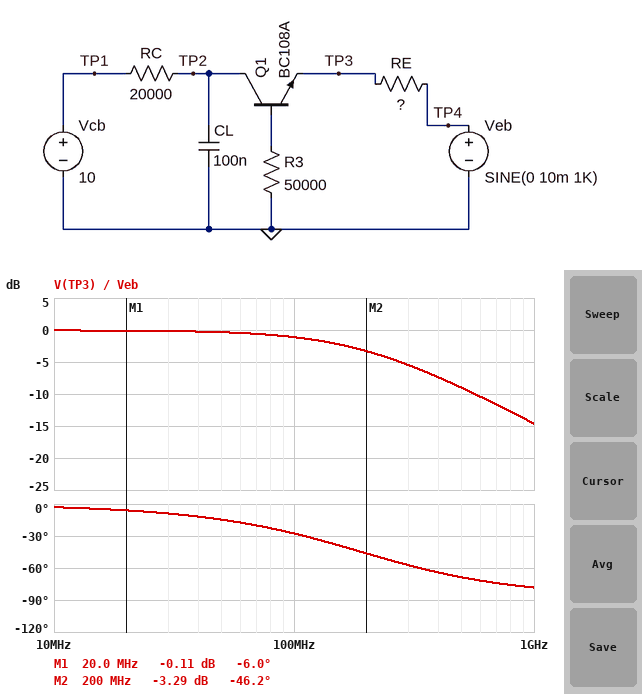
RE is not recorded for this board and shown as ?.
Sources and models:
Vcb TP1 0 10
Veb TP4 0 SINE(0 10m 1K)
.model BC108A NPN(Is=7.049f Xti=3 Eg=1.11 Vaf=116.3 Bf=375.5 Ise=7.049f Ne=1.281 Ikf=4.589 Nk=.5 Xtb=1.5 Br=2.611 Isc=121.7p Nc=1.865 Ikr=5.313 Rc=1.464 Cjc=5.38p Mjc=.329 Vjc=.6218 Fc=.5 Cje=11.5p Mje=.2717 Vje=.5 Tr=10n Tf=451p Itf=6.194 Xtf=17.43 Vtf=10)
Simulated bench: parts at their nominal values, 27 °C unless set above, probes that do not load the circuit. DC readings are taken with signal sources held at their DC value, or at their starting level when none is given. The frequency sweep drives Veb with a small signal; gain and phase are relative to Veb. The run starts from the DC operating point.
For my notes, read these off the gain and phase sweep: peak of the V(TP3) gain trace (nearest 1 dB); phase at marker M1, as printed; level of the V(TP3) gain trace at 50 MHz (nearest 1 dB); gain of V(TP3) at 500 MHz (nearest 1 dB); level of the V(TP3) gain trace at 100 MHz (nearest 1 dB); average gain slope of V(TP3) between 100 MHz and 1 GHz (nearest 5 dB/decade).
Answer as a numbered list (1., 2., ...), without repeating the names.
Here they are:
1. 0 dB
2. -6.0 deg
3. 0 dB
4. -9 dB
5. -1 dB
6. -15 dB/decade
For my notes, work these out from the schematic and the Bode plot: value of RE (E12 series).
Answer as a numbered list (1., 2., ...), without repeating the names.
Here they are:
1. 470 Ω
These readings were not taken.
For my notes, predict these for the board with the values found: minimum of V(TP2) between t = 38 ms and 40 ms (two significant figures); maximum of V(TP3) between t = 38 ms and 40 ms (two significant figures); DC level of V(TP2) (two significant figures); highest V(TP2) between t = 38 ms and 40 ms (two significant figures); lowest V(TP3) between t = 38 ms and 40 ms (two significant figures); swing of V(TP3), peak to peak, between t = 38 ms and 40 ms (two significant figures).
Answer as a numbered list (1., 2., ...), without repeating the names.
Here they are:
1. 10 V
2. 10 mV
3. 10 V
4. 10 V
5. -10 mV
6. 20 mV
